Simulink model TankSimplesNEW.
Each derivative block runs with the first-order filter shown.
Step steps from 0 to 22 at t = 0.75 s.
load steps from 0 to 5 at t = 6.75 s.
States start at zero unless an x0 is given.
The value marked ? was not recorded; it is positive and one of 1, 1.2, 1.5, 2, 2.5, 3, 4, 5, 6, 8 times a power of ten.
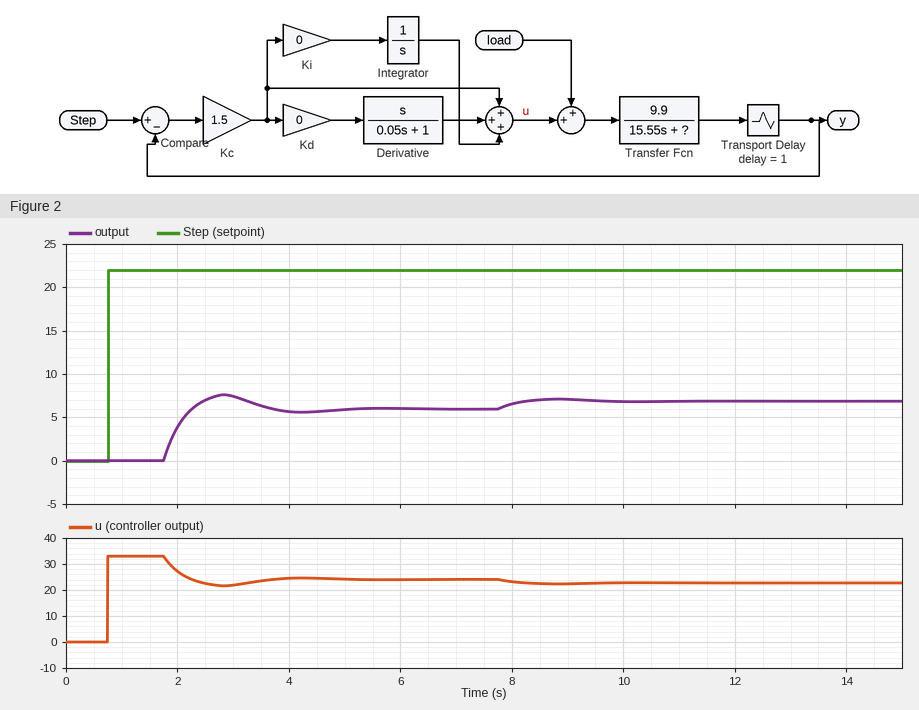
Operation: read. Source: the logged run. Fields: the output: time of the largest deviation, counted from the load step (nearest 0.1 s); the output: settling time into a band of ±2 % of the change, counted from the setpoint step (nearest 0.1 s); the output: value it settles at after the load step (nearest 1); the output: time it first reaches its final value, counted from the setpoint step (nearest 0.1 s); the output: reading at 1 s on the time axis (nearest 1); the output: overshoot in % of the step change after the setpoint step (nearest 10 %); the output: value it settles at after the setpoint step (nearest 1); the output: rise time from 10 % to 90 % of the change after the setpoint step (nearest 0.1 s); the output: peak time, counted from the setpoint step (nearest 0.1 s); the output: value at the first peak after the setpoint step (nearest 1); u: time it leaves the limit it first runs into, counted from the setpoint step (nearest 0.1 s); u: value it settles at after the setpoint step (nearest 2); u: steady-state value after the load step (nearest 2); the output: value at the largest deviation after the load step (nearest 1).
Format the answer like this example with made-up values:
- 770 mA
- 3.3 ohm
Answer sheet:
- 2.1 s
- 4.1 s
- 7
- 1.5 s
- 0
- 30 %
- 6
- 0.4 s
- 2.1 s
- 8
- 1.0 s
- 24
- 22
- 7
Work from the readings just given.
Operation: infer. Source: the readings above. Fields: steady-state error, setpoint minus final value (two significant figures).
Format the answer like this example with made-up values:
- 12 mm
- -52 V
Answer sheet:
- 16
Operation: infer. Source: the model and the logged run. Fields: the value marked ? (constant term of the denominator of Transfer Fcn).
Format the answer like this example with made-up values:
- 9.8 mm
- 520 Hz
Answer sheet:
- 40
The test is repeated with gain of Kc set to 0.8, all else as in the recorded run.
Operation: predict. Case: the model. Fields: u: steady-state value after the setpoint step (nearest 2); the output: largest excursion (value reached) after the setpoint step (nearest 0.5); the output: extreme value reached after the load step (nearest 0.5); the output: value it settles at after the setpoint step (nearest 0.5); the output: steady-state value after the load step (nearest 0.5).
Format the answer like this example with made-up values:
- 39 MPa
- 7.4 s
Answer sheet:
- 14
- 4.0
- 5.0
- 3.5
- 4.5
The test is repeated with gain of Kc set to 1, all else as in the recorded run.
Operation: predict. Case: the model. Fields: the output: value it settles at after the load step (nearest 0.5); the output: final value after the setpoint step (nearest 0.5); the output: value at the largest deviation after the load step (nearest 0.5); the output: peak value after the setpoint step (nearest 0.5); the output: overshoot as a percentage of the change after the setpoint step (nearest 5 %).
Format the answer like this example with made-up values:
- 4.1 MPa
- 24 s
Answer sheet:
- 5.5
- 4.5
- 5.5
- 5.0
- 15 %
